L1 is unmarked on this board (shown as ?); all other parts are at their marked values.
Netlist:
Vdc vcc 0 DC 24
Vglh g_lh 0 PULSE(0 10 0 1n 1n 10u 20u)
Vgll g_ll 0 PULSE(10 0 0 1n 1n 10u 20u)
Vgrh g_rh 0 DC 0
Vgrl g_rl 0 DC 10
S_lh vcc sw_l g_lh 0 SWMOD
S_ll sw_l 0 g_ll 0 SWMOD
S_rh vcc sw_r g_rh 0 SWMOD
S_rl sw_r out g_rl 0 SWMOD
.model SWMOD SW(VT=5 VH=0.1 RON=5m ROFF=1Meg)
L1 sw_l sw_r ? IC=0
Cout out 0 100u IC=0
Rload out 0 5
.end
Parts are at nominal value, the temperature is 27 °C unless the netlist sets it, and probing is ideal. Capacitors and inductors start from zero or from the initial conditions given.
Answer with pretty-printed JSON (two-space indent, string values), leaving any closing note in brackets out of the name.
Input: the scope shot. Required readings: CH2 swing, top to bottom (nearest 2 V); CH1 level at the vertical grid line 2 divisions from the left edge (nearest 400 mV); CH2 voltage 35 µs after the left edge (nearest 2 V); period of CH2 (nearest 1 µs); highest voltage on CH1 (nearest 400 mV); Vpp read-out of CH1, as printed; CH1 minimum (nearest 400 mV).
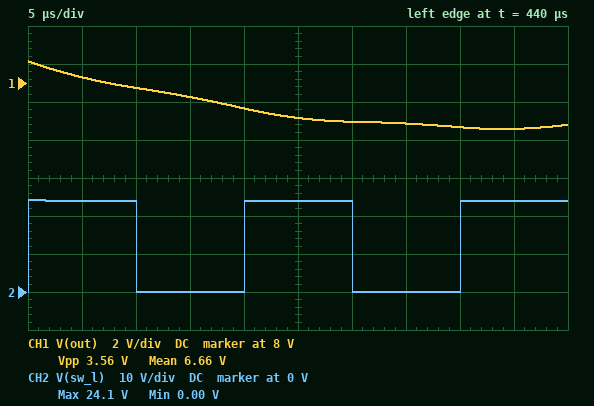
{
  "CH2 swing, top to bottom": "24 V",
  "CH1 level at the vertical grid line 2 divisions from the left edge": "7.6 V",
  "CH2 voltage 35 µs after the left edge": "0 V",
  "period of CH2": "20 µs",
  "highest voltage on CH1": "9.2 V",
  "Vpp read-out of CH1, as printed": "3.56 V",
  "CH1 minimum": "5.6 V"
}
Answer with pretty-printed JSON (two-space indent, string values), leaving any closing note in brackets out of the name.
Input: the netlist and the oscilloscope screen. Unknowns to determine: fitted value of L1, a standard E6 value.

{
  "fitted value of L1, a standard E6 value": "15 µH"
}
